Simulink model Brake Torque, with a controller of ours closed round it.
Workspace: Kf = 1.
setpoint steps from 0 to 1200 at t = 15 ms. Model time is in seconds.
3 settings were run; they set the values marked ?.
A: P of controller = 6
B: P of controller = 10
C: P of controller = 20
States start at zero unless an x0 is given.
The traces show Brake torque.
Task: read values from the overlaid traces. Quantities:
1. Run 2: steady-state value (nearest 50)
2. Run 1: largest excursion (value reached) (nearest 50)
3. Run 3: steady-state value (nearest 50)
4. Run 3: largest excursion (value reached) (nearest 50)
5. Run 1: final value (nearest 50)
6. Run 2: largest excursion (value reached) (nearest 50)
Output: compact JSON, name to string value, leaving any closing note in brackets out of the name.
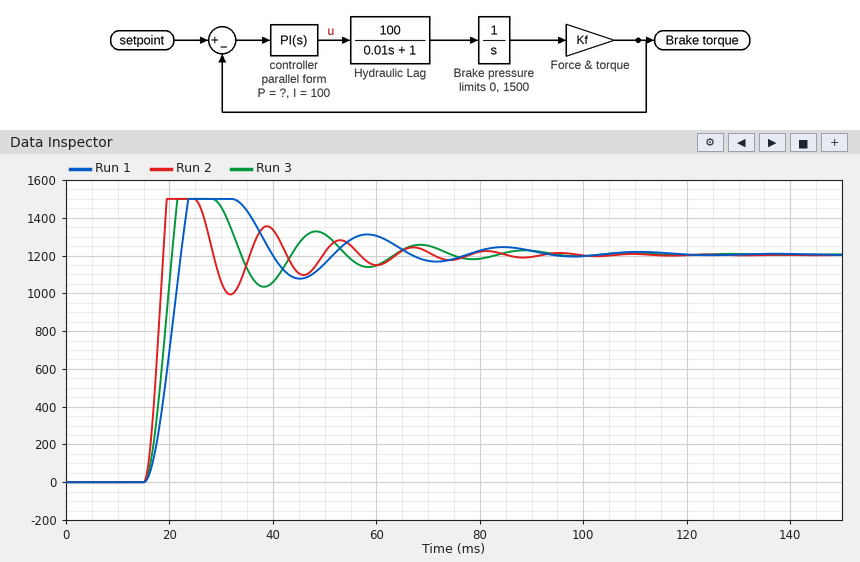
{"Run 2: steady-state value": "1200", "Run 1: largest excursion (value reached)": "1500", "Run 3: steady-state value": "1200", "Run 3: largest excursion (value reached)": "1500", "Run 1: final value": "1200", "Run 2: largest excursion (value reached)": "1500"}
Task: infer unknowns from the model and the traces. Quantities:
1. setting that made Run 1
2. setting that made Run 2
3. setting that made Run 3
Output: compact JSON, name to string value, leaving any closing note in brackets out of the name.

{"setting that made Run 1": "A", "setting that made Run 2": "C", "setting that made Run 3": "B"}
